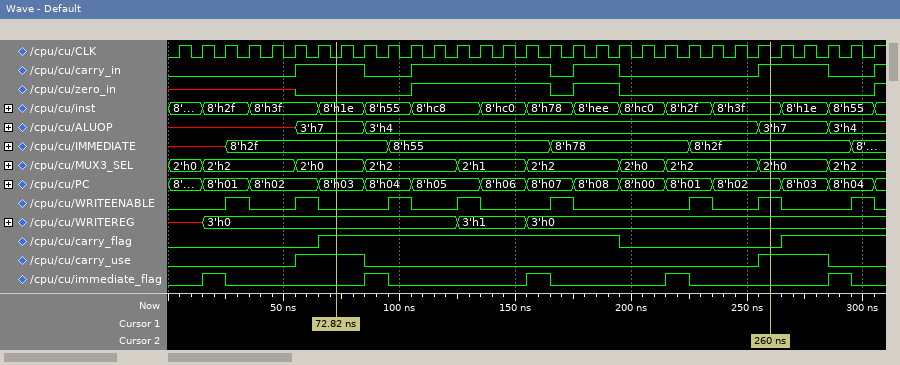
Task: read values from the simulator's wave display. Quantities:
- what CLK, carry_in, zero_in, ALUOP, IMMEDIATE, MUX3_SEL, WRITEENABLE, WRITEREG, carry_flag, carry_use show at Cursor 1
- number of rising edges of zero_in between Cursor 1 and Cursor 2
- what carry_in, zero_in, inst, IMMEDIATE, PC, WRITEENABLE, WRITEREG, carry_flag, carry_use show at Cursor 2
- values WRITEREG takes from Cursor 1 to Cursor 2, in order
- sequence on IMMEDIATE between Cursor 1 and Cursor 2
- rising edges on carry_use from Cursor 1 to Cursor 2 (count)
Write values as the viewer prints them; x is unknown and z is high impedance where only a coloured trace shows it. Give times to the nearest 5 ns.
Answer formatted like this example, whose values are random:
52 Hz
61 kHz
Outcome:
CLK=0, carry_in=1, zero_in=0, ALUOP=3'h7, IMMEDIATE=8'h2f, MUX3_SEL=2'h0, WRITEENABLE=0, WRITEREG=3'h0, carry_flag=1, carry_use=1
2
carry_in=1, zero_in=0, inst=8'h3f, IMMEDIATE=8'h2f, PC=8'h02, WRITEENABLE=1, WRITEREG=3'h0, carry_flag=0, carry_use=1
3'h0, 3'h1, 3'h0
8'h2f, 8'h55, 8'h78, 8'h2f
1
